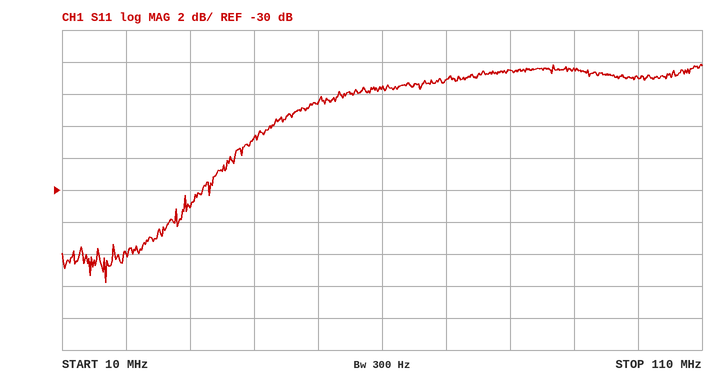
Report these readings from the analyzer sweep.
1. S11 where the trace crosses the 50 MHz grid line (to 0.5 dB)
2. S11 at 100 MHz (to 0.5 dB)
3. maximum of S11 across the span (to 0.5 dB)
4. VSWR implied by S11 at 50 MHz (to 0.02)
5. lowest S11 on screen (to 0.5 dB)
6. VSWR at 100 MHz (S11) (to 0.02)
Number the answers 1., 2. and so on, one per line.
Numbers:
1. -24.5 dB
2. -23.0 dB
3. -22.0 dB
4. 1.12
5. -36.0 dB
6. 1.16
